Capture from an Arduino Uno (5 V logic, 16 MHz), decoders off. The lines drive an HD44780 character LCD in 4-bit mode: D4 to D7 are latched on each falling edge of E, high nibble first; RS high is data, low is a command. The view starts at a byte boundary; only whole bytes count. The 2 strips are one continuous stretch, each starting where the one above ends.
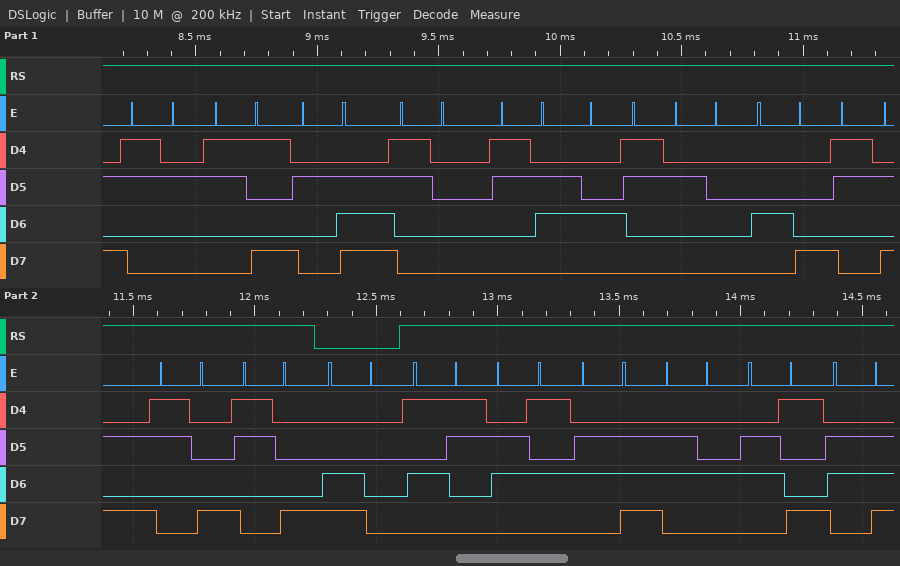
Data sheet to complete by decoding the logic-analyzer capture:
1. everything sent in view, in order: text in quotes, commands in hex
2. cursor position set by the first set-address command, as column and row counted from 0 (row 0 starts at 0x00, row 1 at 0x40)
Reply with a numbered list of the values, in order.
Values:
1. "29.06C H:88" 0xC0 "Sendin"
2. column 0, row 1
